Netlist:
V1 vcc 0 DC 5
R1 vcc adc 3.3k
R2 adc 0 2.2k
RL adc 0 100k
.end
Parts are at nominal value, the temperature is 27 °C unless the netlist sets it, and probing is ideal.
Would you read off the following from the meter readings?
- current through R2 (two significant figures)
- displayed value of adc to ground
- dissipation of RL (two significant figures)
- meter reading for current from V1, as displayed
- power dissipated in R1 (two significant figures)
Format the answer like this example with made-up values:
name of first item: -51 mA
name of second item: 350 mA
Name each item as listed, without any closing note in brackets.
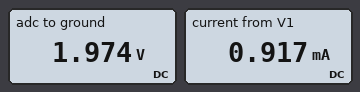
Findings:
current through R2: 900 µA
displayed value of adc to ground: 1.974 V
dissipation of RL: 39 µW
meter reading for current from V1, as displayed: 0.917 mA
power dissipated in R1: 2.8 mW
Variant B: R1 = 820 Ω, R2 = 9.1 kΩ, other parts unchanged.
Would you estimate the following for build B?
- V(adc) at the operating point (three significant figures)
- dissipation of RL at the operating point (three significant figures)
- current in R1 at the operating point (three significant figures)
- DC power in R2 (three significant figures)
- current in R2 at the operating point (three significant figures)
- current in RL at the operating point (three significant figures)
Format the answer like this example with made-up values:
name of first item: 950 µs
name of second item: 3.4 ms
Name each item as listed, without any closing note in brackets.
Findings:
V(adc) at the operating point: 4.55 V
dissipation of RL at the operating point: 207 µW
current in R1 at the operating point: 546 µA
DC power in R2: 2.28 mW
current in R2 at the operating point: 500 µA
current in RL at the operating point: 45.5 µA
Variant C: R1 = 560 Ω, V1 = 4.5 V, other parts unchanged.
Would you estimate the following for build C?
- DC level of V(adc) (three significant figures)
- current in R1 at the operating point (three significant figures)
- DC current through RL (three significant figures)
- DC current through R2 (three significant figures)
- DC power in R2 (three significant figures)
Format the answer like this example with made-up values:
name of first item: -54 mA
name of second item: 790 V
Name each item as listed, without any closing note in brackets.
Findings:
DC level of V(adc): 3.57 V
current in R1 at the operating point: 1.66 mA
DC current through RL: 35.7 µA
DC current through R2: 1.62 mA
DC power in R2: 5.80 mW
